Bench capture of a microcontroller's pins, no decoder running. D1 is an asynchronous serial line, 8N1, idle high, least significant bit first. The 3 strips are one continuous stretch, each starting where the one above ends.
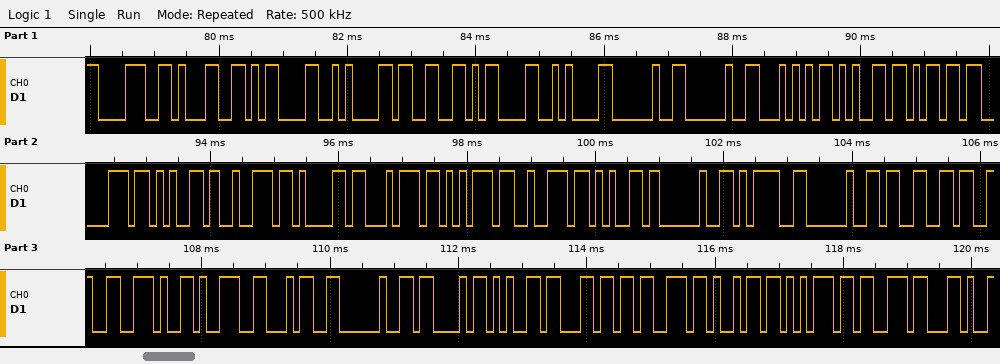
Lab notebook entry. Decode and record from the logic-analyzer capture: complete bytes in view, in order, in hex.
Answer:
38 31 0D 0A 33 0D 0A 20 20 54 65 6D 70 65 72 61 74 75 72 65 20 3D 20 33 33 2E 39 34 20 43 65 6C 73 69 75 73 2C
